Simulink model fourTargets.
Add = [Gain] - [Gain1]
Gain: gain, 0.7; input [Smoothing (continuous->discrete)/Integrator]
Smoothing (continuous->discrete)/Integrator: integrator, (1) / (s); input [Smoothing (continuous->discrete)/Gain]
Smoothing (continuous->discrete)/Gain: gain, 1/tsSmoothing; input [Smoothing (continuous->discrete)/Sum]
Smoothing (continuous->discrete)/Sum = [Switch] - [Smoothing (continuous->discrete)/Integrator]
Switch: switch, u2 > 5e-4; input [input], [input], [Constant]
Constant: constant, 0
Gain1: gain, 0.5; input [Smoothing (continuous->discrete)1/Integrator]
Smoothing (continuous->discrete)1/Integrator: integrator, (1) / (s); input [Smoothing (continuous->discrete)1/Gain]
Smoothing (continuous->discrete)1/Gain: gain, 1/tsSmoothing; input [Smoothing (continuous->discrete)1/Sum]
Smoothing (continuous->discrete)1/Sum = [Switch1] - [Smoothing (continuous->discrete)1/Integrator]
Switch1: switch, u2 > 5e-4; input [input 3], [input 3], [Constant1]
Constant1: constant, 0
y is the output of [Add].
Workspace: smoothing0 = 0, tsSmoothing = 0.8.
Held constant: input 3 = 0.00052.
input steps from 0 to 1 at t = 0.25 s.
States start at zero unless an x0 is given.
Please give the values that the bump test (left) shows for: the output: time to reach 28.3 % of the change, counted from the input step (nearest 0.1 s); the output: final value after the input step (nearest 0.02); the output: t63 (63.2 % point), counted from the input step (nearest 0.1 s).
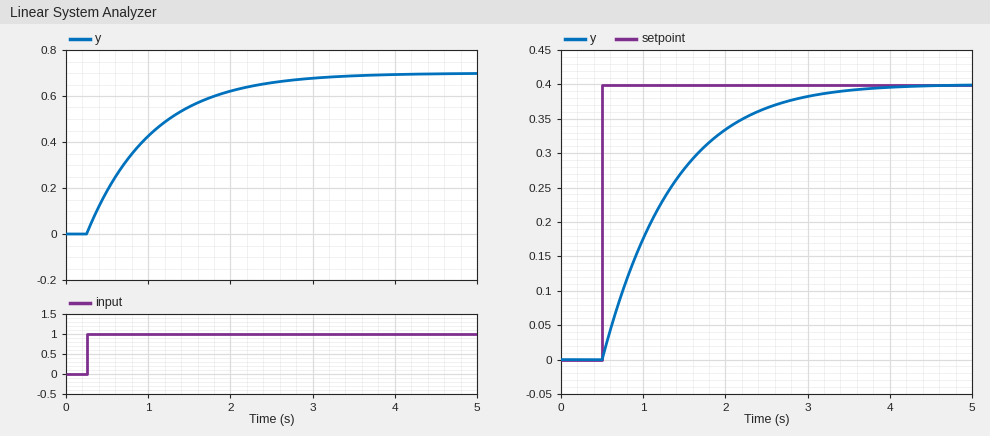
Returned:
0.3 s
0.70
0.8 s
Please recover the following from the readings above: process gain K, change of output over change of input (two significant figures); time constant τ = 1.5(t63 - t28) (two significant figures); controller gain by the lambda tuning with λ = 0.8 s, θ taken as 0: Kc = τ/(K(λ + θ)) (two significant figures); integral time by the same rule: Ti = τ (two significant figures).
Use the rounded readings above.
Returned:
0.70
0.75 s
1.3
0.75 s
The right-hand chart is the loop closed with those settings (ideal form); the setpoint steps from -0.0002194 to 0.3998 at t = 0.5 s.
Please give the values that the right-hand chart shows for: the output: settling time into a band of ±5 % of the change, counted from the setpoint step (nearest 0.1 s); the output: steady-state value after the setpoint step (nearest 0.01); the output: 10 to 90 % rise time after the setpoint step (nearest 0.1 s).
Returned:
2.4 s
0.40
1.8 s
